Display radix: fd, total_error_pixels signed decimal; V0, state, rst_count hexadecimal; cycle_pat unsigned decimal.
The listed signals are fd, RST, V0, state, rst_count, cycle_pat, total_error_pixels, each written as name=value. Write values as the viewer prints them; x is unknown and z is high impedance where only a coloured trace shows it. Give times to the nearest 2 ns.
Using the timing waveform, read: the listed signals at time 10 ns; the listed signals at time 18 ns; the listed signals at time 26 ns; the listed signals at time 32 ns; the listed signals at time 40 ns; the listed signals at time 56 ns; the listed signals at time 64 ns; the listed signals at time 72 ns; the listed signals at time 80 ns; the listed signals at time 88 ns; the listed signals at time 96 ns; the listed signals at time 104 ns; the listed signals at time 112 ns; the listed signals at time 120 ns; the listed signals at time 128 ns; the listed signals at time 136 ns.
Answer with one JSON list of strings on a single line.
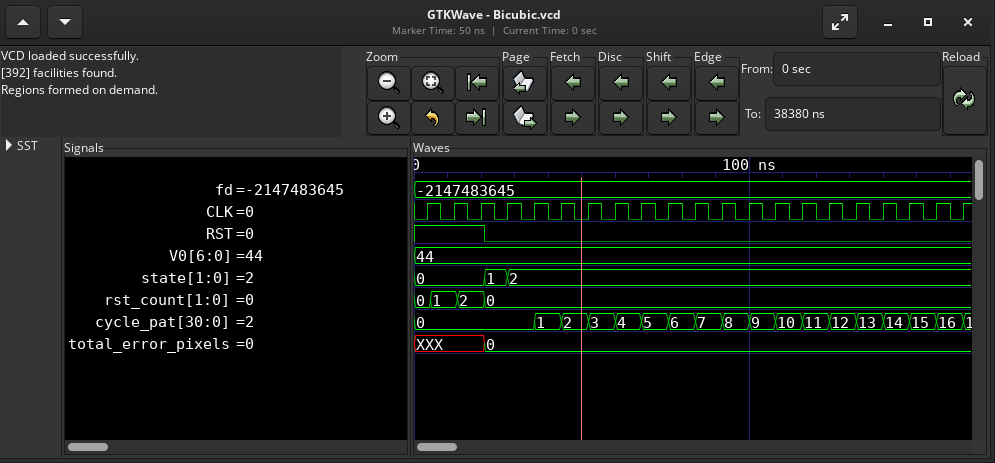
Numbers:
["fd=-2147483645, RST=1, V0=44, state=0, rst_count=1, cycle_pat=0, total_error_pixels=XXX", "fd=-2147483645, RST=1, V0=44, state=0, rst_count=2, cycle_pat=0, total_error_pixels=XXX", "fd=-2147483645, RST=0, V0=44, state=1, rst_count=0, cycle_pat=0, total_error_pixels=0", "fd=-2147483645, RST=0, V0=44, state=2, rst_count=0, cycle_pat=0, total_error_pixels=0", "fd=-2147483645, RST=0, V0=44, state=2, rst_count=0, cycle_pat=1, total_error_pixels=0", "fd=-2147483645, RST=0, V0=44, state=2, rst_count=0, cycle_pat=3, total_error_pixels=0", "fd=-2147483645, RST=0, V0=44, state=2, rst_count=0, cycle_pat=4, total_error_pixels=0", "fd=-2147483645, RST=0, V0=44, state=2, rst_count=0, cycle_pat=5, total_error_pixels=0", "fd=-2147483645, RST=0, V0=44, state=2, rst_count=0, cycle_pat=6, total_error_pixels=0", "fd=-2147483645, RST=0, V0=44, state=2, rst_count=0, cycle_pat=7, total_error_pixels=0", "fd=-2147483645, RST=0, V0=44, state=2, rst_count=0, cycle_pat=8, total_error_pixels=0", "fd=-2147483645, RST=0, V0=44, state=2, rst_count=0, cycle_pat=9, total_error_pixels=0", "fd=-2147483645, RST=0, V0=44, state=2, rst_count=0, cycle_pat=10, total_error_pixels=0", "fd=-2147483645, RST=0, V0=44, state=2, rst_count=0, cycle_pat=11, total_error_pixels=0", "fd=-2147483645, RST=0, V0=44, state=2, rst_count=0, cycle_pat=12, total_error_pixels=0", "fd=-2147483645, RST=0, V0=44, state=2, rst_count=0, cycle_pat=13, total_error_pixels=0"]
